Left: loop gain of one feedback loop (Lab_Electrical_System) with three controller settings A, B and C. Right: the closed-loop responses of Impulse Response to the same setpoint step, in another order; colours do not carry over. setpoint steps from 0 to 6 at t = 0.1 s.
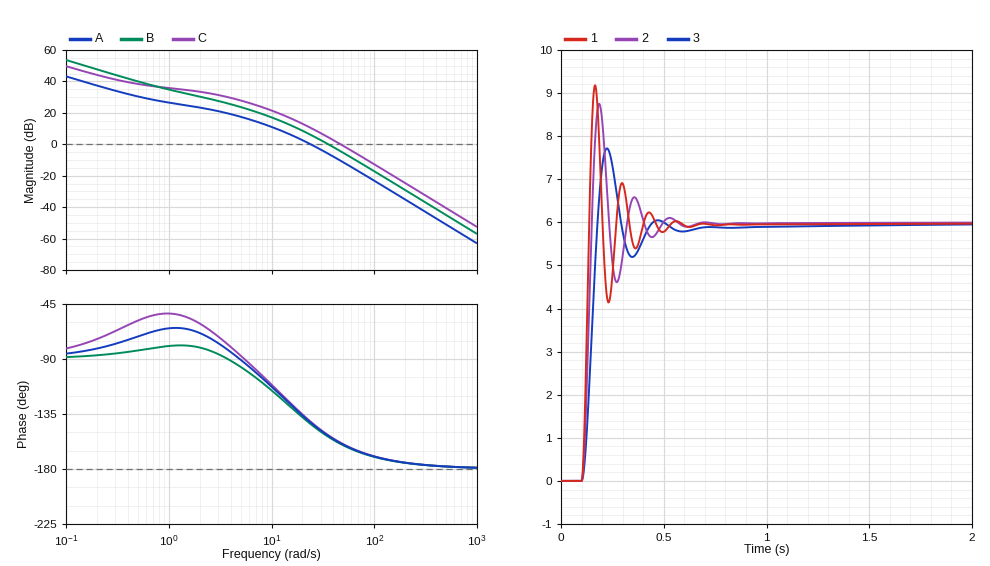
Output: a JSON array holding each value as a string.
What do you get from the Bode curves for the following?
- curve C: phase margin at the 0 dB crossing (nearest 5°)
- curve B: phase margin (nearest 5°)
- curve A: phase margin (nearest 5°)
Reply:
["20°", "25°", "40°"]
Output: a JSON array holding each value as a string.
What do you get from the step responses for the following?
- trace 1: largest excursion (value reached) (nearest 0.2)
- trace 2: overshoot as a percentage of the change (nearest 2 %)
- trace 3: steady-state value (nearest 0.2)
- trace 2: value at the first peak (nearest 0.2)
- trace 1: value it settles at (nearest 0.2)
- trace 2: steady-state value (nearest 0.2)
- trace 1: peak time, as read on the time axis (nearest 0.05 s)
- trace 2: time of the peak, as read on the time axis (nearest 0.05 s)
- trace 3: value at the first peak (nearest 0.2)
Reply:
["9.2", "46 %", "6.0", "8.8", "6.0", "6.0", "0.15 s", "0.20 s", "7.8"]
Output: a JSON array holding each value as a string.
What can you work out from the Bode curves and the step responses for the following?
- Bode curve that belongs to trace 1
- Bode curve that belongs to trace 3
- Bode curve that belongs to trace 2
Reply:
["C", "A", "B"]
